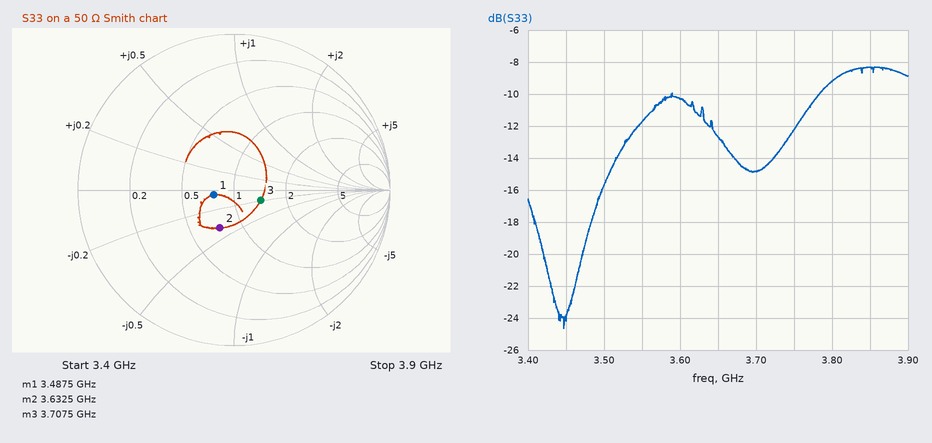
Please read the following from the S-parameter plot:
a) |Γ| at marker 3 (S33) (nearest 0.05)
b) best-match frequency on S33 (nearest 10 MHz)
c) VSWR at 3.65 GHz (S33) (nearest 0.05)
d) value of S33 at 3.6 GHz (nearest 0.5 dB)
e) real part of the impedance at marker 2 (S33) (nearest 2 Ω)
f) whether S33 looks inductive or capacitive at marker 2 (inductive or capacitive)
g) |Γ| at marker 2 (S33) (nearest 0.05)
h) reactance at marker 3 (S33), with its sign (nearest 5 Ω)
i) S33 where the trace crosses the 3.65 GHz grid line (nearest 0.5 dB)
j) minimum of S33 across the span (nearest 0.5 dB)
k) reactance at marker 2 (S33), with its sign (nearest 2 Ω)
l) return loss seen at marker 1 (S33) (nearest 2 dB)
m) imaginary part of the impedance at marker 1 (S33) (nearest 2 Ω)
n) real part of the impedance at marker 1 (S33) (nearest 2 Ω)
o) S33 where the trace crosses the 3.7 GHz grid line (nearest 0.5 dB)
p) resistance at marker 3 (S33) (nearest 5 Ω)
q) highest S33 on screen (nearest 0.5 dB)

0.20
3.45 GHz
1.60
-10.5 dB
38 Ω
capacitive
0.25
-10 Ω
-12.5 dB
-24.5 dB
-20 Ω
18 dB
-2 Ω
38 Ω
-15.0 dB
70 Ω
-8.5 dB
